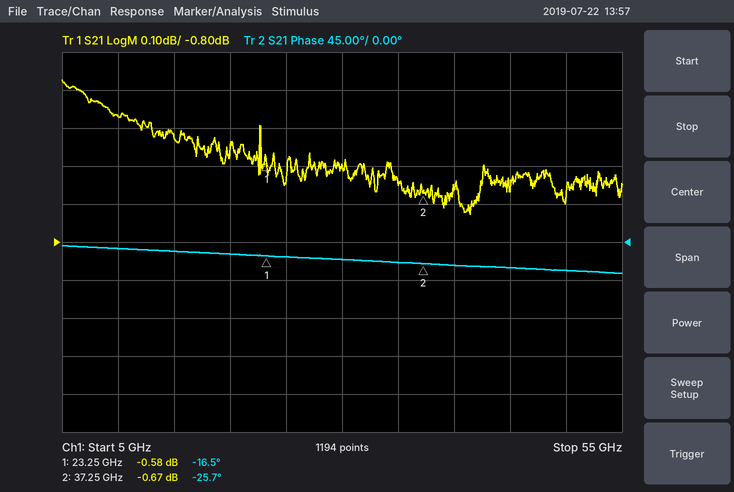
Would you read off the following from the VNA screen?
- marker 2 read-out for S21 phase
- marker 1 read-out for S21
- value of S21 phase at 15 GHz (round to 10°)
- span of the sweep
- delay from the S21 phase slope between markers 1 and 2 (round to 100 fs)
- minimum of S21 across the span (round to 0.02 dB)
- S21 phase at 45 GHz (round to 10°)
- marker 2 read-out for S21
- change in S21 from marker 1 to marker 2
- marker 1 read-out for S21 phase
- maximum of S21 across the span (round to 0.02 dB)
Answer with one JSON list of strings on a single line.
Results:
["-25.7°", "-0.58 dB", "-10°", "50 GHz", "1.8 ps", "-0.72 dB", "-30°", "-0.67 dB", "-0.09 dB", "-16.5°", "-0.38 dB"]
